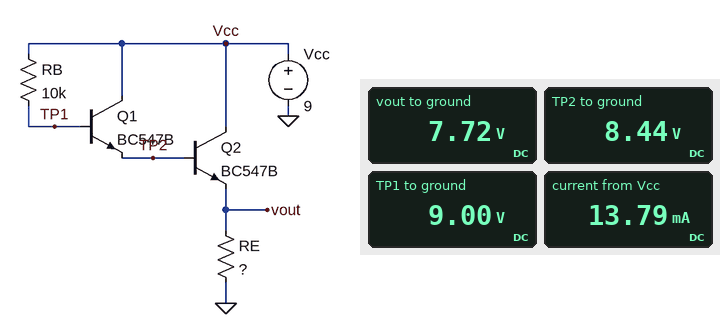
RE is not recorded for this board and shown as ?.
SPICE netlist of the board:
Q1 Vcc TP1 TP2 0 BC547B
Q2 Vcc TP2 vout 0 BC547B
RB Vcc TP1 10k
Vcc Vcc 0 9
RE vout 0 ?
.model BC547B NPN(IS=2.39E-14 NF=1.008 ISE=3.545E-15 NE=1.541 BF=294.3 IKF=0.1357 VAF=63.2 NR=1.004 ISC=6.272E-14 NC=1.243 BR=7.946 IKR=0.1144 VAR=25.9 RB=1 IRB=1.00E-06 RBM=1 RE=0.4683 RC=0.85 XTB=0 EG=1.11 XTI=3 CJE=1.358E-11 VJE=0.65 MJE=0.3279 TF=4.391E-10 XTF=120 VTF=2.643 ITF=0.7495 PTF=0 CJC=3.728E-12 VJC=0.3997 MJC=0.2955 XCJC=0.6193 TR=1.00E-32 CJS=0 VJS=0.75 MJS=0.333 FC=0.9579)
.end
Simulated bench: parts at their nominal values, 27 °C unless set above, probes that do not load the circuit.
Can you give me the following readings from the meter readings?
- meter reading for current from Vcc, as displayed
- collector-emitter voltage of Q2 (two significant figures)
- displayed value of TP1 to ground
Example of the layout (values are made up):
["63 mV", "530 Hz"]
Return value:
["13.79 mA", "1.3 V", "9.00 V"]
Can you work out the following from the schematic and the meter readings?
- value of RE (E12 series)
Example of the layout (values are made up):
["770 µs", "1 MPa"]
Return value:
["560 Ω"]
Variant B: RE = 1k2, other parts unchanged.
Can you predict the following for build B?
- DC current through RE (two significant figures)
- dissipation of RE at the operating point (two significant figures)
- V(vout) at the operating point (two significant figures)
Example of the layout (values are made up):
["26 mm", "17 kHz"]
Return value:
["6.5 mA", "50 mW", "7.8 V"]
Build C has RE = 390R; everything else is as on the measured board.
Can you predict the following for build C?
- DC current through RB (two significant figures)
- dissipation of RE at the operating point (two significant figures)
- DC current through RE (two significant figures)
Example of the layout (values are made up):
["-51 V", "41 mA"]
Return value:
["280 nA", "150 mW", "20 mA"]
